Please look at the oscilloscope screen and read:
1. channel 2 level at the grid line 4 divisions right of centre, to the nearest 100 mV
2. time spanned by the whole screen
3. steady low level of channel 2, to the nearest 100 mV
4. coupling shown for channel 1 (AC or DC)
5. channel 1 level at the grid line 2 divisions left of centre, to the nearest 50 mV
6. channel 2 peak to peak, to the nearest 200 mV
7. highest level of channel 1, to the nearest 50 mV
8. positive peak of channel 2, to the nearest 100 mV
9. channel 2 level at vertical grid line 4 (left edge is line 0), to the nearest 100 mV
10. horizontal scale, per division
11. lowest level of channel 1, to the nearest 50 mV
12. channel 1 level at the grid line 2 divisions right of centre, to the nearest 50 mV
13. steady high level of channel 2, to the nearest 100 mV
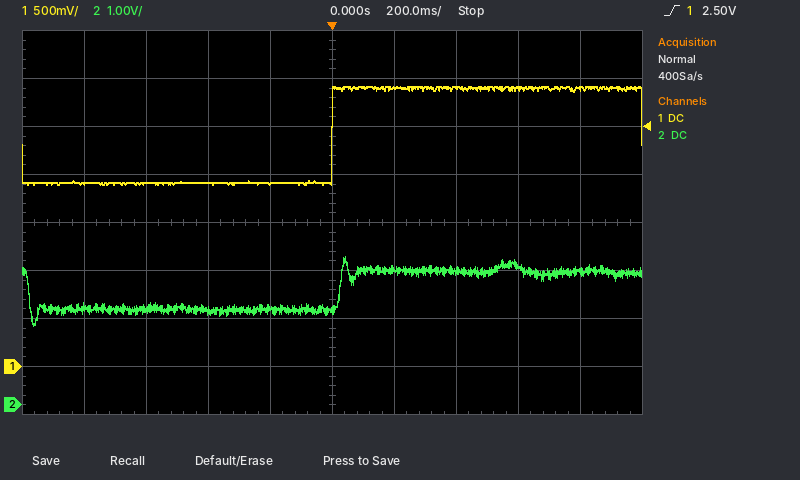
2.8 V
2 s
2.0 V
DC
1.90 V
1.4 V
2.90 V
3.1 V
2.0 V
200 ms
1.90 V
2.90 V
2.8 V
